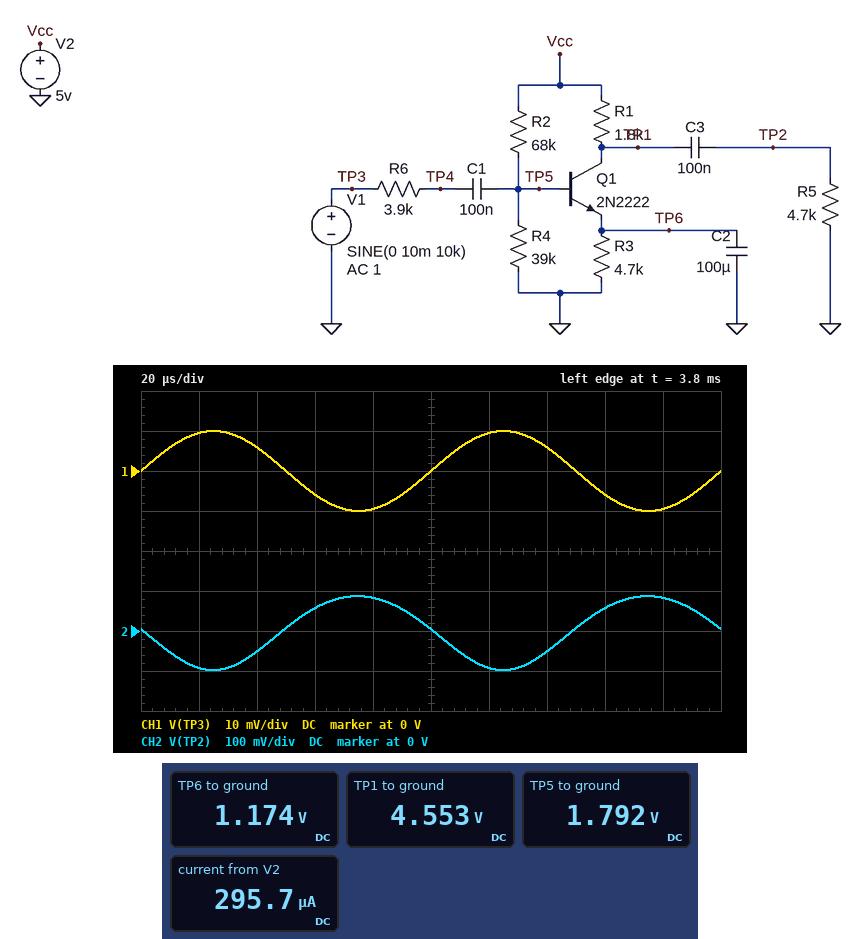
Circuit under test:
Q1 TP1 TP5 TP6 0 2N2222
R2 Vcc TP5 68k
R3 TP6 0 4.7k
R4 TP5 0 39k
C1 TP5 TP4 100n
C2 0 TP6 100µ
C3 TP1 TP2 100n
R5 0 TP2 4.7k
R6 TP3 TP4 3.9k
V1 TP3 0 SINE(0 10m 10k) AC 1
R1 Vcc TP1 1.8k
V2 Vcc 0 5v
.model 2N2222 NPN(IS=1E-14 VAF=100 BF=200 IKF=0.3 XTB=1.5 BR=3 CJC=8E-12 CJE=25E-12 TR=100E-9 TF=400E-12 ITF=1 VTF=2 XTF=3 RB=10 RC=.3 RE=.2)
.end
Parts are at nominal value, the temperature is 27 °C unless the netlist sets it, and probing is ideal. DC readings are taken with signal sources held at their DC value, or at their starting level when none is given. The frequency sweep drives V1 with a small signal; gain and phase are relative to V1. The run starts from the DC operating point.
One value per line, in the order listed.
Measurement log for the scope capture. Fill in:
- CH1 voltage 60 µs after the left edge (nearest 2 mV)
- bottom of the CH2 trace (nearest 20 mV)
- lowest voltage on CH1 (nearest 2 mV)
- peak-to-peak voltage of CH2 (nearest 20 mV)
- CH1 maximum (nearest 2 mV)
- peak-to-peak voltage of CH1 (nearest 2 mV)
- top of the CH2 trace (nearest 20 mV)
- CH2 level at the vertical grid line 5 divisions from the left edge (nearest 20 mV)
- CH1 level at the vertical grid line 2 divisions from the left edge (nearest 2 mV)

-6 mV
-100 mV
-10 mV
180 mV
10 mV
20 mV
80 mV
0 V
6 mV
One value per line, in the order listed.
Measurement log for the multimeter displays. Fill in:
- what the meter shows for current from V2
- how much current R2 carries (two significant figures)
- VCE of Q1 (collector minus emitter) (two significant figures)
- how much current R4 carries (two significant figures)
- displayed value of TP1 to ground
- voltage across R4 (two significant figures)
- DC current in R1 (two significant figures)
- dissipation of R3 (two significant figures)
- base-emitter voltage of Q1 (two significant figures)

295.7 µA
47 µA
3.4 V
46 µA
4.553 V
1.8 V
250 µA
290 µW
620 mV
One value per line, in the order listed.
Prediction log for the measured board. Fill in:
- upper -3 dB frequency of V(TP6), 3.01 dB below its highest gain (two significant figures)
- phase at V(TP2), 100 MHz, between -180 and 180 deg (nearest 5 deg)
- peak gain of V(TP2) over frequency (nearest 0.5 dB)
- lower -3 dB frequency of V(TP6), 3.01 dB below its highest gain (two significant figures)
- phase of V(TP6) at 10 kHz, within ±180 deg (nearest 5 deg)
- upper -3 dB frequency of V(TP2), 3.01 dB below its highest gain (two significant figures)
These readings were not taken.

120 Hz
15 deg
19.5 dB
6.2 Hz
-90 deg
510 kHz
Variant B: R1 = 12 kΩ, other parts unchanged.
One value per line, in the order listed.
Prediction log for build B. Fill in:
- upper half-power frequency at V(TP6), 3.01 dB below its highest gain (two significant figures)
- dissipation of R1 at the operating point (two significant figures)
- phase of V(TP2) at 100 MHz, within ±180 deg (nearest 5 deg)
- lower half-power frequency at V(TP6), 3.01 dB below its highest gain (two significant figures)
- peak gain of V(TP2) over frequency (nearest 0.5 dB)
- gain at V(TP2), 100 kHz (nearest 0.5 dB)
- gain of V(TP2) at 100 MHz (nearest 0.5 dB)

130 Hz
740 µW
0 deg
6.0 Hz
27.5 dB
26.5 dB
-34.0 dB
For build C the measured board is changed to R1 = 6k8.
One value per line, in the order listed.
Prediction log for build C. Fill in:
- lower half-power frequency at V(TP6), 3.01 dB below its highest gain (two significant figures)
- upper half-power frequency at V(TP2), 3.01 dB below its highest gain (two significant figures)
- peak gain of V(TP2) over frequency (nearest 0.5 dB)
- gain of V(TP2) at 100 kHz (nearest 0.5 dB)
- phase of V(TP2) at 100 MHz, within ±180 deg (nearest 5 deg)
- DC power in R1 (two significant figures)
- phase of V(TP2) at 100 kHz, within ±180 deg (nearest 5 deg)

6.1 Hz
280 kHz
26.0 dB
25.5 dB
5 deg
420 µW
160 deg
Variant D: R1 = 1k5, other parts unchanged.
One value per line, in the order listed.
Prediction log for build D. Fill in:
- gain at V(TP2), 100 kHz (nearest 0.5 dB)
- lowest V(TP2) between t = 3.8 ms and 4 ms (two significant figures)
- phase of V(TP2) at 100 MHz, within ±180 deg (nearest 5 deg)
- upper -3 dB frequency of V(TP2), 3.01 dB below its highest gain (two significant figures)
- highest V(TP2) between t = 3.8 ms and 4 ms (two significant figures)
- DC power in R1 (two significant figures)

18.0 dB
-86 mV
20 deg
550 kHz
76 mV
93 µW
